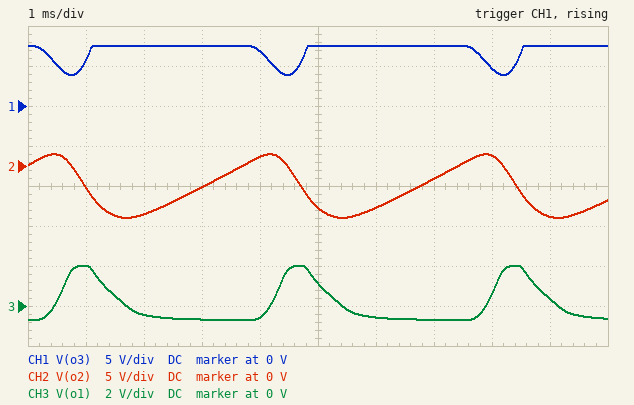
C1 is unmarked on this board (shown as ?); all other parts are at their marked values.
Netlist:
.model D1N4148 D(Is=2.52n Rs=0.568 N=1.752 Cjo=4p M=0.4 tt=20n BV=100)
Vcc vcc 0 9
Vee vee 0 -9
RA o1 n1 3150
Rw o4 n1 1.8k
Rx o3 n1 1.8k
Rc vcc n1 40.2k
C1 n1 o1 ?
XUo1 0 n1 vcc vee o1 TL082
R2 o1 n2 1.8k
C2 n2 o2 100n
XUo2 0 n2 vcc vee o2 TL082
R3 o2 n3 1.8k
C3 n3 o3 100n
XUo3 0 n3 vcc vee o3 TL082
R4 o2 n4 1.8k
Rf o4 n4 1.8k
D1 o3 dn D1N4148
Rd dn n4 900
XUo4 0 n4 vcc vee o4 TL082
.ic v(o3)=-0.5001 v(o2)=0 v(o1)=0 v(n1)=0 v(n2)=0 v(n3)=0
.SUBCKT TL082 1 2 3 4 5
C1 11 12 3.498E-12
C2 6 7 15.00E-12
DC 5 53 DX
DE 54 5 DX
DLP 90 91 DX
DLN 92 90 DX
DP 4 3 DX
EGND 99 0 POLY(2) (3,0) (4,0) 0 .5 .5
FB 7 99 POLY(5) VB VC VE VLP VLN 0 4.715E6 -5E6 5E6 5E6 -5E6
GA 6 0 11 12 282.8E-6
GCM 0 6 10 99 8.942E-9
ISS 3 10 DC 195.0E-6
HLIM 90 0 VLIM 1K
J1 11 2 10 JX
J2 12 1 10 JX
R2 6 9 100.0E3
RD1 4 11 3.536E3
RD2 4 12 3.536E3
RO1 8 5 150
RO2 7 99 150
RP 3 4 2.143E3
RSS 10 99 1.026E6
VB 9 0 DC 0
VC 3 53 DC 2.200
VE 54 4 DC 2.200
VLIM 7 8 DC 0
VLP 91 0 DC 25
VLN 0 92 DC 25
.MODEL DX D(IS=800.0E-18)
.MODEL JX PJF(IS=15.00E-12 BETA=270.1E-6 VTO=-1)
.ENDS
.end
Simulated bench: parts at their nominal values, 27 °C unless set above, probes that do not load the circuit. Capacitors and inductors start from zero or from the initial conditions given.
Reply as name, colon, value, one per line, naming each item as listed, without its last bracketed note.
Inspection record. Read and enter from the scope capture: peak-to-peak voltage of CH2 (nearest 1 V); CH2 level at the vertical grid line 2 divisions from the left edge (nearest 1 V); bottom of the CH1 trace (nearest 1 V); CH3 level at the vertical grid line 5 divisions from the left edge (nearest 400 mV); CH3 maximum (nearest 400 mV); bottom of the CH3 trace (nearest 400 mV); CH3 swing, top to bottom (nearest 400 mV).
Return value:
peak-to-peak voltage of CH2: 8 V
CH2 level at the vertical grid line 2 divisions from the left edge: -6 V
bottom of the CH1 trace: 4 V
CH3 level at the vertical grid line 5 divisions from the left edge: 1.2 V
CH3 maximum: 2.0 V
bottom of the CH3 trace: -800 mV
CH3 swing, top to bottom: 2.8 V
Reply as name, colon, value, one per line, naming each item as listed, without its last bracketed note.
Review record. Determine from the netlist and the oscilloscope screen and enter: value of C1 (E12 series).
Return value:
value of C1: 180 nF
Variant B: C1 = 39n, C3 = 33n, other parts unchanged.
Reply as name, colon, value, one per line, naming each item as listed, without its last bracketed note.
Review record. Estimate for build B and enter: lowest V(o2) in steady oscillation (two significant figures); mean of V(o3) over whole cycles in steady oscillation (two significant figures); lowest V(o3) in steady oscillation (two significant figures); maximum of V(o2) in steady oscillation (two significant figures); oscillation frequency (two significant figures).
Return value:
lowest V(o2) in steady oscillation: -1.9 V
mean of V(o3) over whole cycles in steady oscillation: 7.1 V
lowest V(o3) in steady oscillation: 5.5 V
maximum of V(o2) in steady oscillation: 570 mV
oscillation frequency: 820 Hz
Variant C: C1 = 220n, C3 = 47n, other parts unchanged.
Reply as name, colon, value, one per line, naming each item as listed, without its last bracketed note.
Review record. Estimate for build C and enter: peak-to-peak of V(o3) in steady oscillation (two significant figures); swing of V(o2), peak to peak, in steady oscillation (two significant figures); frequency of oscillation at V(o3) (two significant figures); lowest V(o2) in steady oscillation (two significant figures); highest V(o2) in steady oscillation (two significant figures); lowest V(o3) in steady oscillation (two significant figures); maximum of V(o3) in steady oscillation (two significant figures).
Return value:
peak-to-peak of V(o3) in steady oscillation: 4.5 V
swing of V(o2), peak to peak, in steady oscillation: 6.0 V
frequency of oscillation at V(o3): 280 Hz
lowest V(o2) in steady oscillation: -5.0 V
highest V(o2) in steady oscillation: 1.0 V
lowest V(o3) in steady oscillation: 2.9 V
maximum of V(o3) in steady oscillation: 7.5 V
